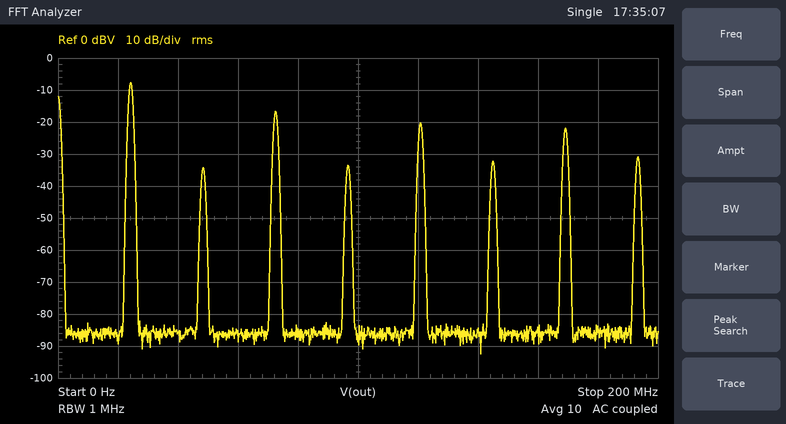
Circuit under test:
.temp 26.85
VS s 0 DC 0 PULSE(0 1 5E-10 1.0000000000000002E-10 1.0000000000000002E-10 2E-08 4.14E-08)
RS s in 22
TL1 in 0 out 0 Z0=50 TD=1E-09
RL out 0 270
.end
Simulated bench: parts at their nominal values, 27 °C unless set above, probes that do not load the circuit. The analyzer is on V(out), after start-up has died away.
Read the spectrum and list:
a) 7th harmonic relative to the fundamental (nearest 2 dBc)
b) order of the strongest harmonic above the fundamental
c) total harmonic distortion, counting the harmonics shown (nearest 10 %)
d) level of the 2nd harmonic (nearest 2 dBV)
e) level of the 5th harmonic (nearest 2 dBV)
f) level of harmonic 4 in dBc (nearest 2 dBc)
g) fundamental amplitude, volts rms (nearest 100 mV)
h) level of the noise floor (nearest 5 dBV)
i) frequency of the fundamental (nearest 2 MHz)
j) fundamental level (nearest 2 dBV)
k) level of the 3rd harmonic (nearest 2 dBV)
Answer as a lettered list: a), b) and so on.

a) -14 dBc
b) 3
c) 50 %
d) -34 dBV
e) -20 dBV
f) -26 dBc
g) 400 mV
h) -85 dBV
i) 24 MHz
j) -8 dBV
k) -16 dBV
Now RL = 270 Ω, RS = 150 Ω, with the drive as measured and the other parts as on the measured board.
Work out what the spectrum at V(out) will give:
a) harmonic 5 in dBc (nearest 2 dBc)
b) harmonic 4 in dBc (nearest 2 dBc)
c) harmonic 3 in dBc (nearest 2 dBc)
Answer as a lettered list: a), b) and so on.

a) -18 dBc
b) -30 dBc
c) -12 dBc
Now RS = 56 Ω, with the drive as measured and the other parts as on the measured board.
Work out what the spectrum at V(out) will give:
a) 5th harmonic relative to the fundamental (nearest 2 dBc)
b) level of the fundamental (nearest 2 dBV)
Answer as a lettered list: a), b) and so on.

a) -14 dBc
b) -8 dBV
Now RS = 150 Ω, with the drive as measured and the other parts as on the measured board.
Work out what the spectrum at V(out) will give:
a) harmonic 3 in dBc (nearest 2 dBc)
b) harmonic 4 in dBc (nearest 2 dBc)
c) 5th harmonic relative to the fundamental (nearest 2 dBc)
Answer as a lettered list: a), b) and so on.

a) -12 dBc
b) -30 dBc
c) -18 dBc
